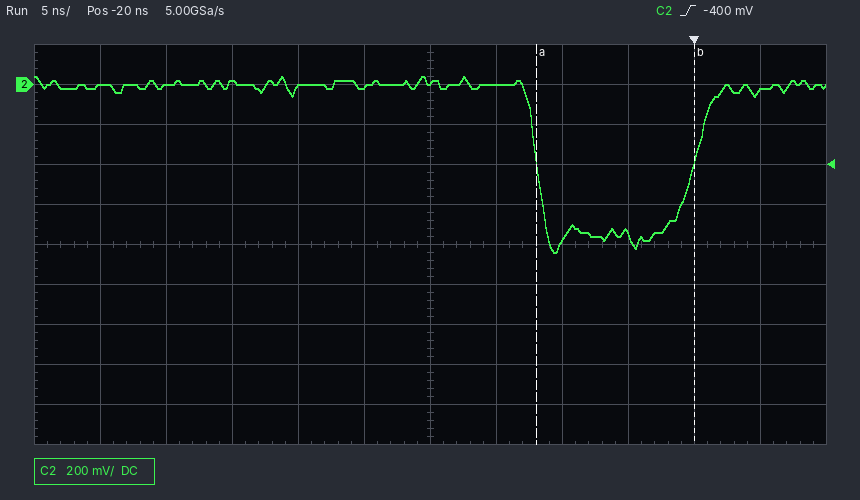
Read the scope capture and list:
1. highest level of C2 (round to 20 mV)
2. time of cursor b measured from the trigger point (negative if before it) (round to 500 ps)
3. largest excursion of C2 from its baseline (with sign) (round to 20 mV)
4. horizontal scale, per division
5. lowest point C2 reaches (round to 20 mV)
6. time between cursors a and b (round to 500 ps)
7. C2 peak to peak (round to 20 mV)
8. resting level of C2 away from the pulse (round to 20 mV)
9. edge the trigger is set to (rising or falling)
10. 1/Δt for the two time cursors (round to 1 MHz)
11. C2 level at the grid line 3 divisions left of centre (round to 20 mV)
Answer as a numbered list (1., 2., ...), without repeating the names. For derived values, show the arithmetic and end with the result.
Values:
1. 40 mV
2. 0.0 ns
3. -840 mV − (0 mV) = -840 mV
4. 5 ns
5. -840 mV
6. 12.0 ns
7. 40 mV − (-840 mV) = 880 mV
8. 0 mV
9. rising
10. 1 / 12.0 ns ≈ 83 MHz
11. 20 mV
